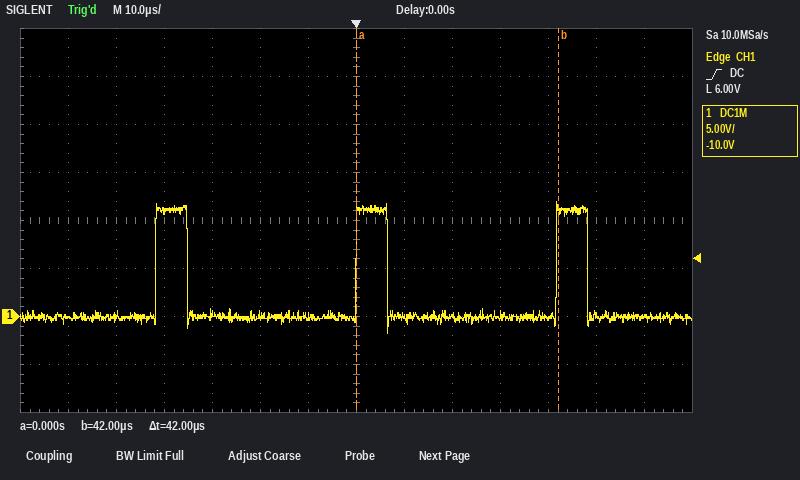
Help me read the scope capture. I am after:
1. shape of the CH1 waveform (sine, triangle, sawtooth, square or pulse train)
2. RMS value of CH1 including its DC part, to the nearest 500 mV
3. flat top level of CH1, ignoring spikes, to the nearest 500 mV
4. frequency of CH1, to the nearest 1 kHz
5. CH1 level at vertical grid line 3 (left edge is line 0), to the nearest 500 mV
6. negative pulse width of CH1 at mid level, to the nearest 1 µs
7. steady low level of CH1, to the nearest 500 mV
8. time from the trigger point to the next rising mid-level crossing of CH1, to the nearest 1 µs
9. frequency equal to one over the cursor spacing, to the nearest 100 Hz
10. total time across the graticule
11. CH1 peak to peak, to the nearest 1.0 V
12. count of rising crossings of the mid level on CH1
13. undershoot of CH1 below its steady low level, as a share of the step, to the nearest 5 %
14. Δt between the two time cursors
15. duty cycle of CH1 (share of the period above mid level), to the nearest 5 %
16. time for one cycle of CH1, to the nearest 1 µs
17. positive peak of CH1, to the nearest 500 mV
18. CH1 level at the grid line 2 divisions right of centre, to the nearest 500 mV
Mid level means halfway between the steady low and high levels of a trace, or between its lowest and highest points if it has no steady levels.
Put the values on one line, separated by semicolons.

pulse train; 4.5 V; 11.0 V; 24 kHz; 11.0 V; 35 µs; 0.0 V; 42 µs; 23.8 kHz; 140 µs; 14.0 V; 3; 15 %; 42 µs; 15 %; 42 µs; 12.0 V; 0.0 V
